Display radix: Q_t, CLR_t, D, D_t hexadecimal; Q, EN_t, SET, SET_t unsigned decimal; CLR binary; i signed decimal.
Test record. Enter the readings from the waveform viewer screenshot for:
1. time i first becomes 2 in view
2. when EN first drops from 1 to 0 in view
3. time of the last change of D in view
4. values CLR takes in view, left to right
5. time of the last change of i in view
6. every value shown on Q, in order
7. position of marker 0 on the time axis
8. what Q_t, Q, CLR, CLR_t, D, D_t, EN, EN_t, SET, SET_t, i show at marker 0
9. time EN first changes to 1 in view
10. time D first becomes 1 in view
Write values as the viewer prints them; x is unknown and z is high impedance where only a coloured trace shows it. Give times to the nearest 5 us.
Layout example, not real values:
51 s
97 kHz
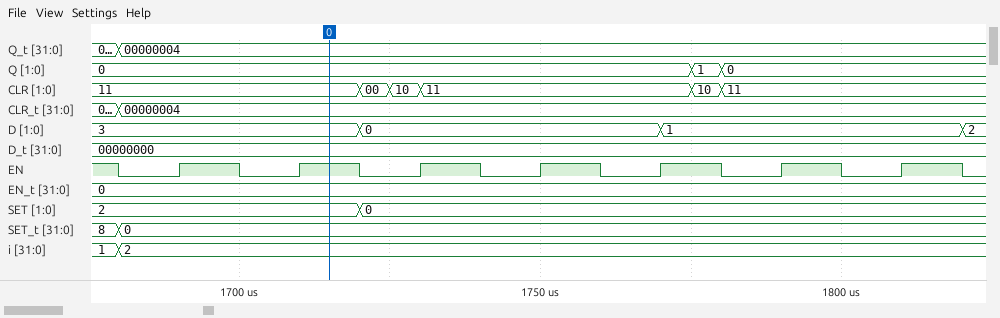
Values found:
1680 us
1680 us
1820 us
11, 00, 10, 11, 10, 11
1680 us
0, 1, 0
1715 us
Q_t=00000004, Q=0, CLR=11, CLR_t=00000004, D=3, D_t=00000000, EN=1, EN_t=0, SET=2, SET_t=0, i=2
1690 us
1770 us
